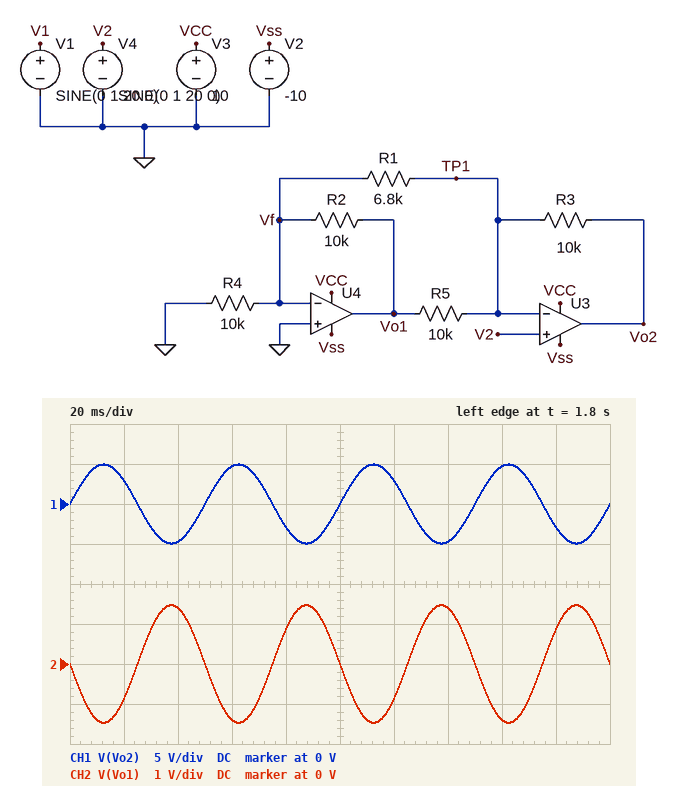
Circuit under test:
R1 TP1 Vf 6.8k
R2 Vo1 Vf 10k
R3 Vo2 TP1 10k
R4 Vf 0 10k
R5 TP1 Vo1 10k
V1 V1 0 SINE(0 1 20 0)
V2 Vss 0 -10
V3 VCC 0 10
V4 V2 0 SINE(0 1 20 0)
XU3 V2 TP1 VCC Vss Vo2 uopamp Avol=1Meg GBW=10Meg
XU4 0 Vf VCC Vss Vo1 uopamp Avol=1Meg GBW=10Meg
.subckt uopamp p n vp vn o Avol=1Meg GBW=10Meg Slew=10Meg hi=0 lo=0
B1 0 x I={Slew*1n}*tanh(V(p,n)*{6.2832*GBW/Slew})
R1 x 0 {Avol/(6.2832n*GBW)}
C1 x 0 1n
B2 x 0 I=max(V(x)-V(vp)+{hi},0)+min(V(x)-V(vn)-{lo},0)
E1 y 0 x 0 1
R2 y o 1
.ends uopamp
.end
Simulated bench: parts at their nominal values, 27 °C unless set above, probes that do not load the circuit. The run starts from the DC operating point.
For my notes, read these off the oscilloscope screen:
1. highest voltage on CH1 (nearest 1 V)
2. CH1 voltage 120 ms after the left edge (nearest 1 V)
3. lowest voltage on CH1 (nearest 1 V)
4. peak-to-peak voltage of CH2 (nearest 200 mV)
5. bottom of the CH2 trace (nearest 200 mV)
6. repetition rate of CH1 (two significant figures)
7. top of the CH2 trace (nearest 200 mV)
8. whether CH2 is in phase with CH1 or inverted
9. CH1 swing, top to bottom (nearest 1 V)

5 V
3 V
-5 V
3.0 V
-1.4 V
20 Hz
1.4 V
inverted
10 V
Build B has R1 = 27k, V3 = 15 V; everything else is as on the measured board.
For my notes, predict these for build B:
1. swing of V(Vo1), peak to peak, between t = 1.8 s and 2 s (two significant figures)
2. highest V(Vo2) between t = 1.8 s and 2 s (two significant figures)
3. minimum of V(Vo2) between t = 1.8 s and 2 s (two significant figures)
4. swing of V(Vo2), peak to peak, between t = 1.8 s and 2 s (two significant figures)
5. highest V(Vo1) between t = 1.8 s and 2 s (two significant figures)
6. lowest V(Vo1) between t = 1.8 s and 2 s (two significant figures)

740 mV
2.7 V
-2.7 V
5.5 V
370 mV
-370 mV
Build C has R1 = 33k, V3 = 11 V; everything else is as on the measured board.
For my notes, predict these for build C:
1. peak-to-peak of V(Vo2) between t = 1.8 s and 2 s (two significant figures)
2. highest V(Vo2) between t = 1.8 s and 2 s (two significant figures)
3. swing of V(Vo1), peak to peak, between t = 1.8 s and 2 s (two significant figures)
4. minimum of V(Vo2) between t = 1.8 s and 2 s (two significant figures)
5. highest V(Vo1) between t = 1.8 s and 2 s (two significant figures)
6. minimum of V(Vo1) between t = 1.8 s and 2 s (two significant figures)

5.2 V
2.6 V
610 mV
-2.6 V
300 mV
-300 mV
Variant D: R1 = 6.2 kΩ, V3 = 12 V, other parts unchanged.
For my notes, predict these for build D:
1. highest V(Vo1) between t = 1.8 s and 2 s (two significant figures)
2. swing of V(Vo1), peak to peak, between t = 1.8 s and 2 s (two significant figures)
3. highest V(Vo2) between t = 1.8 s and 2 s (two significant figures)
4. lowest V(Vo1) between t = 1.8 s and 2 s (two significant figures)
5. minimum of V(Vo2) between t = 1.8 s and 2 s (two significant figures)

1.6 V
3.2 V
5.2 V
-1.6 V
-5.2 V
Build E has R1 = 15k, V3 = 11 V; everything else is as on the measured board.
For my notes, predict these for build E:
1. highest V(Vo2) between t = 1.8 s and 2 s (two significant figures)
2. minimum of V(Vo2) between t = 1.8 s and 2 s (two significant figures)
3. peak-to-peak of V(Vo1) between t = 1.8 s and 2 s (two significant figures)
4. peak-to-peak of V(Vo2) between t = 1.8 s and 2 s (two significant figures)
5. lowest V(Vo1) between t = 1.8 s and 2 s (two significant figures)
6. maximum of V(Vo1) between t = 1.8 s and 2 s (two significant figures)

3.3 V
-3.3 V
1.3 V
6.7 V
-670 mV
670 mV
